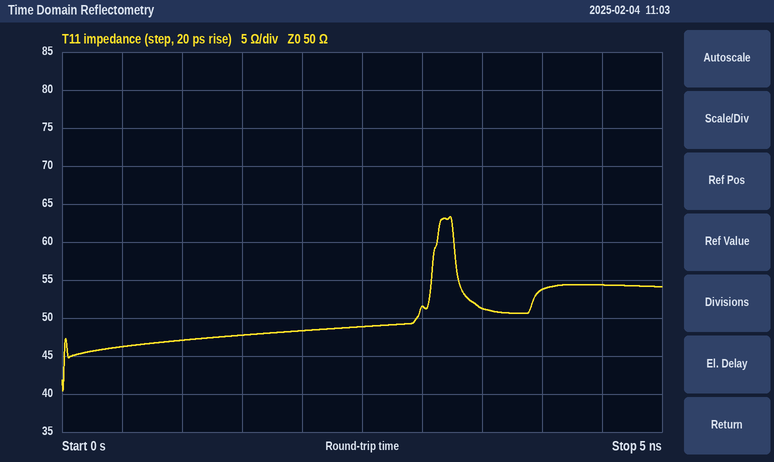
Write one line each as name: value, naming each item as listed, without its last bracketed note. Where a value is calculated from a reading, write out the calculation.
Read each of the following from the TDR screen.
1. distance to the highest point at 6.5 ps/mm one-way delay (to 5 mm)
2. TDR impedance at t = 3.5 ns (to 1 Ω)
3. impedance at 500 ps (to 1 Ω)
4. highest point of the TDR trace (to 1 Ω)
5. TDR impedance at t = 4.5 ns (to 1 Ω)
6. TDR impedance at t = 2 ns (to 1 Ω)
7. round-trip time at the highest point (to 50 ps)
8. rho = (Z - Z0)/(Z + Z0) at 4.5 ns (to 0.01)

distance to the highest point at 6.5 ps/mm one-way delay: 3.25 ns / 2 / 6.5 ps/mm ≈ 250 mm
TDR impedance at t = 3.5 ns: 51 Ω
impedance at 500 ps: 46 Ω
highest point of the TDR trace: 63 Ω
TDR impedance at t = 4.5 ns: 54 Ω
TDR impedance at t = 2 ns: 48 Ω
round-trip time at the highest point: 3.25 ns
rho = (Z - Z0)/(Z + Z0) at 4.5 ns: (54 − 50)/(54 + 50) ≈ +0.04
